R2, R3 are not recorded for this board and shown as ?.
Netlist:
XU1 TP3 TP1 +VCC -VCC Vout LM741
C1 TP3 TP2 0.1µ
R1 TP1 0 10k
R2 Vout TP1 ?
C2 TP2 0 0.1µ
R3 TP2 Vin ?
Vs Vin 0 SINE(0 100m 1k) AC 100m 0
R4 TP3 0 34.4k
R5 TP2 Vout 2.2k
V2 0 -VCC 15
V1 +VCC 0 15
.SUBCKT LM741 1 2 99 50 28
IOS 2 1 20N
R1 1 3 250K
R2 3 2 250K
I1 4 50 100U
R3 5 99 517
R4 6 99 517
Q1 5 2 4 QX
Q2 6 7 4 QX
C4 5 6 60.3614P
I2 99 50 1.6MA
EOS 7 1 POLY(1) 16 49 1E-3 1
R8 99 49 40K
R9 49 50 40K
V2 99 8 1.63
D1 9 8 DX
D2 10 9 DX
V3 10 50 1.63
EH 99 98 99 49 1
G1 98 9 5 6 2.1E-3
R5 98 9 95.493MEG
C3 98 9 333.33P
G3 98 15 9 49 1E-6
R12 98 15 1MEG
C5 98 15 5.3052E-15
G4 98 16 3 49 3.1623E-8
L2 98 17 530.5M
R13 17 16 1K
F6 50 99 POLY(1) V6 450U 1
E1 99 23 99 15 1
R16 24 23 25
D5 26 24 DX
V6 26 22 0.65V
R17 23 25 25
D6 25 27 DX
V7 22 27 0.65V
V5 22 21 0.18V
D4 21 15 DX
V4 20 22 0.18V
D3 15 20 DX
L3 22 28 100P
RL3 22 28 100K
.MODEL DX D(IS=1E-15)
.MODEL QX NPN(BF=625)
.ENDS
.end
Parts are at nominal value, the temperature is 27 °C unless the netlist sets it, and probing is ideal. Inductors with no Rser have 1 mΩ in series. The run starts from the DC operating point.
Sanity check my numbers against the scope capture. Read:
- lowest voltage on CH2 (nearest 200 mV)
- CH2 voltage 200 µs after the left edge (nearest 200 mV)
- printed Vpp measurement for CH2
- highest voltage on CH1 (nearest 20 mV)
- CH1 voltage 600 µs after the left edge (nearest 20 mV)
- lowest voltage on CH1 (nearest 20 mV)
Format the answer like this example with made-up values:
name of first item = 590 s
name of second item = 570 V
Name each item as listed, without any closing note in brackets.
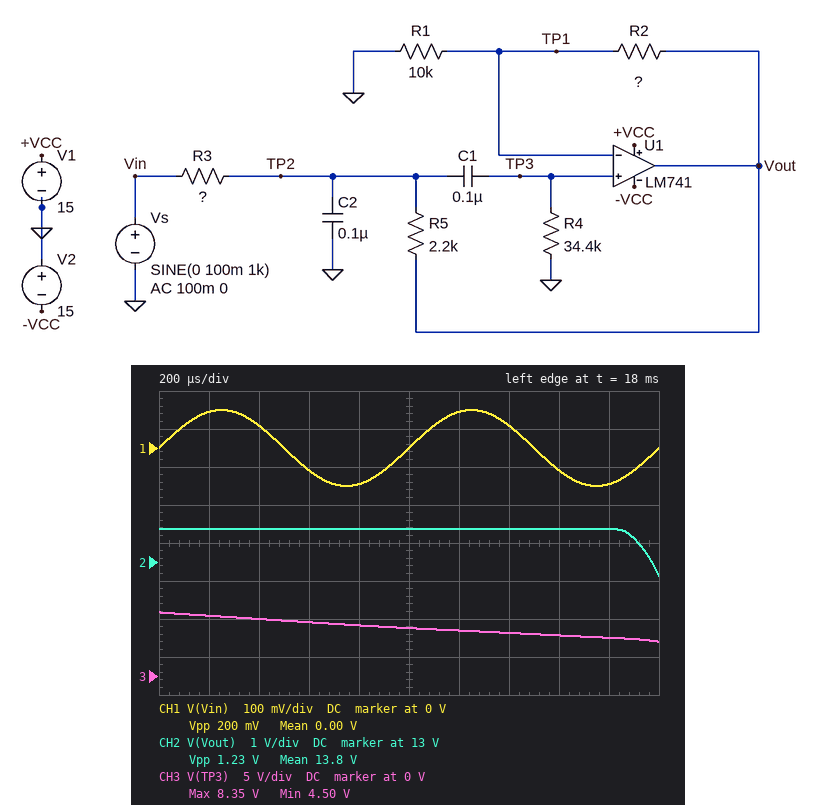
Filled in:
lowest voltage on CH2 = 12.6 V
CH2 voltage 200 µs after the left edge = 13.8 V
printed Vpp measurement for CH2 = 1.23 V
highest voltage on CH1 = 100 mV
CH1 voltage 600 µs after the left edge = -60 mV
lowest voltage on CH1 = -100 mV
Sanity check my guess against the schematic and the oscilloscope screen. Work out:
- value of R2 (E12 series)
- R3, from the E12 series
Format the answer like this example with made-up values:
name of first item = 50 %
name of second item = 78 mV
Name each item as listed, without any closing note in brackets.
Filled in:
value of R2 = 18 kΩ
R3, from the E12 series = 4.7 kΩ
